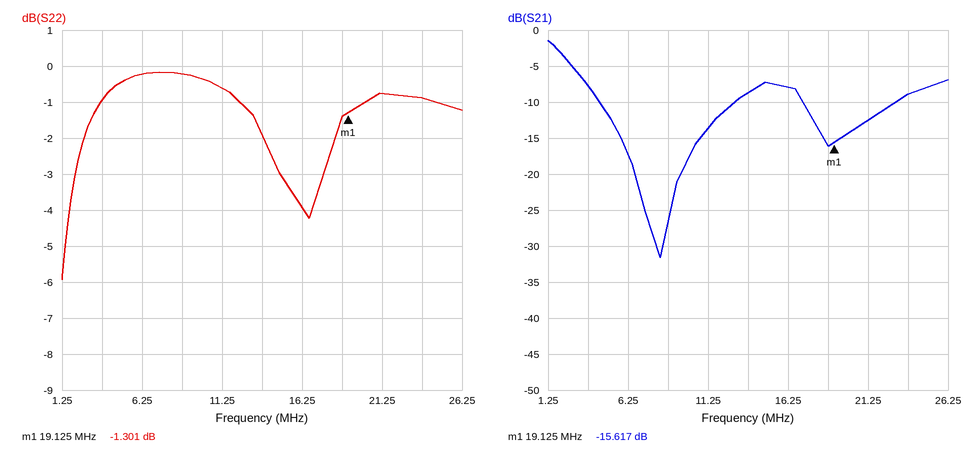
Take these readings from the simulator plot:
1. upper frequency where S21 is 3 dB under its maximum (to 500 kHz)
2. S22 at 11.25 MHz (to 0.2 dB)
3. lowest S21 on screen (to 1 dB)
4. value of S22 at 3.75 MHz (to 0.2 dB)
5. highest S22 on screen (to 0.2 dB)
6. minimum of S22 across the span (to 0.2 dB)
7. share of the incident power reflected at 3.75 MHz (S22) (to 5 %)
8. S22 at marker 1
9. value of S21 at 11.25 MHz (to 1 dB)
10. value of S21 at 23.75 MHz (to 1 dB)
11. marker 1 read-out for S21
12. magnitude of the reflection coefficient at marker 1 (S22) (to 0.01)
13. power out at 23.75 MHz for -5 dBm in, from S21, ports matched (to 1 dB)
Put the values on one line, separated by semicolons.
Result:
2.5 MHz; -0.6 dB; -32 dB; -1.0 dB; -0.2 dB; -6.0 dB; 80 %; -1.301 dB; -14 dB; -9 dB; -15.617 dB; 0.86; -14 dBm
